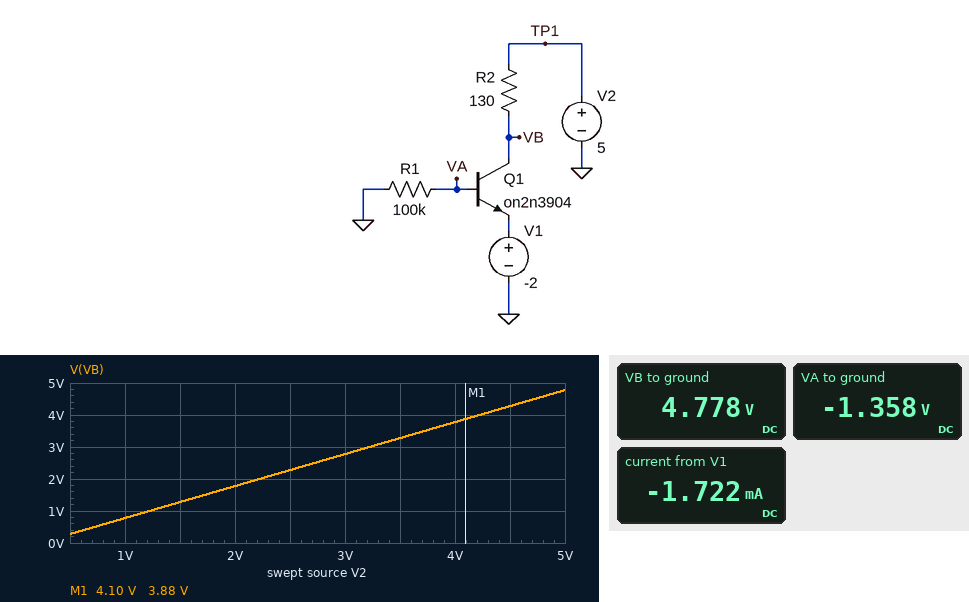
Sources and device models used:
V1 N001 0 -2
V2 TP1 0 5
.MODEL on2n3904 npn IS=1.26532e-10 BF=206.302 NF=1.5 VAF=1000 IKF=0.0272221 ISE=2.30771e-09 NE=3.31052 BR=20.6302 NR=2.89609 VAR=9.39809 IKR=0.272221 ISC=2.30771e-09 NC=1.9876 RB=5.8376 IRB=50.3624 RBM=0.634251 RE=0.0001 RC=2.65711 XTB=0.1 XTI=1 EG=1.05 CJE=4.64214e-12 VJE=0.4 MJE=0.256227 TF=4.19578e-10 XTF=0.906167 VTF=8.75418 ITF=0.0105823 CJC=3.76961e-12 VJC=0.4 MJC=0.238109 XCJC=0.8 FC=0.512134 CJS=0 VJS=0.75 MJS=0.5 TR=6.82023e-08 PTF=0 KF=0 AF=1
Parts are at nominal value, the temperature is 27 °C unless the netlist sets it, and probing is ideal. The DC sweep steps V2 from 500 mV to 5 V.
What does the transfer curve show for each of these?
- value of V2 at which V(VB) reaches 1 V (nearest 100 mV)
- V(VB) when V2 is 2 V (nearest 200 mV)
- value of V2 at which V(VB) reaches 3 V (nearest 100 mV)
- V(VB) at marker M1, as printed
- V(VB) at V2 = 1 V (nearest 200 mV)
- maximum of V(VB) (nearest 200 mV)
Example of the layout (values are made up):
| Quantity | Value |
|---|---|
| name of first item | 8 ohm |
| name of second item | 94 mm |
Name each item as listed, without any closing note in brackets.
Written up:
| Quantity | Value |
|---|---|
| value of V2 at which V(VB) reaches 1 V | 1.2 V |
| V(VB) when V2 is 2 V | 1.8 V |
| value of V2 at which V(VB) reaches 3 V | 3.2 V |
| V(VB) at marker M1, as printed | 3.88 V |
| V(VB) at V2 = 1 V | 800 mV |
| maximum of V(VB) | 4.8 V |
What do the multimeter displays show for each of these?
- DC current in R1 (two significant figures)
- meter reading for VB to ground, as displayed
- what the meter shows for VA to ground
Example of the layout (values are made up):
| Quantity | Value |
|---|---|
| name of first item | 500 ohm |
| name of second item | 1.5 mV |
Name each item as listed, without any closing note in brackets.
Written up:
| Quantity | Value |
|---|---|
| DC current in R1 | 14 µA |
| meter reading for VB to ground, as displayed | 4.778 V |
| what the meter shows for VA to ground | -1.358 V |
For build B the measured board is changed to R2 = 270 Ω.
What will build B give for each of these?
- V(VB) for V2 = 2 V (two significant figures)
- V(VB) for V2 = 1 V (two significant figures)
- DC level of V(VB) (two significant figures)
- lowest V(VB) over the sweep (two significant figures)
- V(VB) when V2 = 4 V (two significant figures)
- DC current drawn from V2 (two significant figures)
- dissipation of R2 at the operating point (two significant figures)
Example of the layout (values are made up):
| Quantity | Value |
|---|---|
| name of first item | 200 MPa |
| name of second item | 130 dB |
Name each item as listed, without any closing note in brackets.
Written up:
| Quantity | Value |
|---|---|
| V(VB) for V2 = 2 V | 1.5 V |
| V(VB) for V2 = 1 V | 540 mV |
| DC level of V(VB) | 4.5 V |
| lowest V(VB) over the sweep | 41 mV |
| V(VB) when V2 = 4 V | 3.5 V |
| DC current drawn from V2 | 1.7 mA |
| dissipation of R2 at the operating point | 790 µW |
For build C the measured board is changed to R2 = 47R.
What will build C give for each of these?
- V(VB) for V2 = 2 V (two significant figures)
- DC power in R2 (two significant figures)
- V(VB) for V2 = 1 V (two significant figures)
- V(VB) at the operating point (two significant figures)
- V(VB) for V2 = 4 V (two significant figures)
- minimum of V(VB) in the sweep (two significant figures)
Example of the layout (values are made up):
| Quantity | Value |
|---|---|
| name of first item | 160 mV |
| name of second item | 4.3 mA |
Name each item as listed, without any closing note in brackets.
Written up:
| Quantity | Value |
|---|---|
| V(VB) for V2 = 2 V | 1.9 V |
| DC power in R2 | 140 µW |
| V(VB) for V2 = 1 V | 920 mV |
| V(VB) at the operating point | 4.9 V |
| V(VB) for V2 = 4 V | 3.9 V |
| minimum of V(VB) in the sweep | 420 mV |
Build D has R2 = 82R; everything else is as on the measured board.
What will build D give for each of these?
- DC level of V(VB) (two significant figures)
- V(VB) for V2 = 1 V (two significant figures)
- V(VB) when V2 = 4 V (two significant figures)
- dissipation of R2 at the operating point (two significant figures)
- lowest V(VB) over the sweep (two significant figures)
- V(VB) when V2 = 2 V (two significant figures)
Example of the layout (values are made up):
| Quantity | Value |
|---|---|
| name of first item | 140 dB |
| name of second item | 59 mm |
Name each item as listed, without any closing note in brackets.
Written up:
| Quantity | Value |
|---|---|
| DC level of V(VB) | 4.9 V |
| V(VB) for V2 = 1 V | 860 mV |
| V(VB) when V2 = 4 V | 3.9 V |
| dissipation of R2 at the operating point | 240 µW |
| lowest V(VB) over the sweep | 360 mV |
| V(VB) when V2 = 2 V | 1.9 V |
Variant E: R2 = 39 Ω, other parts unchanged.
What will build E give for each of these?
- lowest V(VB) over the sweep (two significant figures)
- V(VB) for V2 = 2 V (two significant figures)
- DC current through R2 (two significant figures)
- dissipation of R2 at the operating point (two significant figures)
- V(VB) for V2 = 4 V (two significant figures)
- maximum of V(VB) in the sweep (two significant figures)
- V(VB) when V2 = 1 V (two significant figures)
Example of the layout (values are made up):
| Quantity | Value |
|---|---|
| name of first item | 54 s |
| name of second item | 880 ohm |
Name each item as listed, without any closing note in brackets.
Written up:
| Quantity | Value |
|---|---|
| lowest V(VB) over the sweep | 430 mV |
| V(VB) for V2 = 2 V | 1.9 V |
| DC current through R2 | 1.7 mA |
| dissipation of R2 at the operating point | 110 µW |
| V(VB) for V2 = 4 V | 3.9 V |
| maximum of V(VB) in the sweep | 4.9 V |
| V(VB) when V2 = 1 V | 930 mV |
